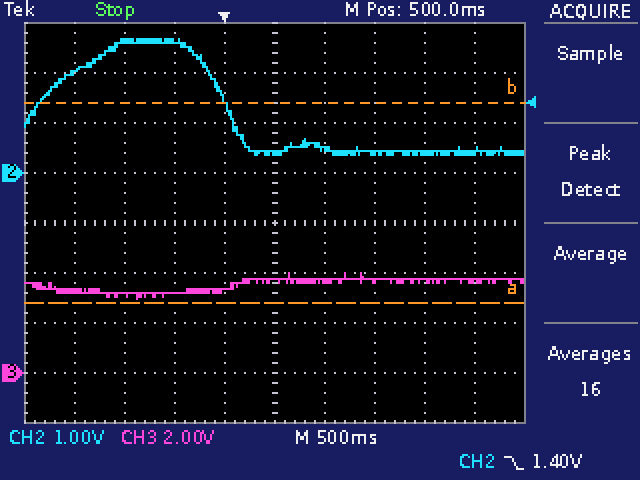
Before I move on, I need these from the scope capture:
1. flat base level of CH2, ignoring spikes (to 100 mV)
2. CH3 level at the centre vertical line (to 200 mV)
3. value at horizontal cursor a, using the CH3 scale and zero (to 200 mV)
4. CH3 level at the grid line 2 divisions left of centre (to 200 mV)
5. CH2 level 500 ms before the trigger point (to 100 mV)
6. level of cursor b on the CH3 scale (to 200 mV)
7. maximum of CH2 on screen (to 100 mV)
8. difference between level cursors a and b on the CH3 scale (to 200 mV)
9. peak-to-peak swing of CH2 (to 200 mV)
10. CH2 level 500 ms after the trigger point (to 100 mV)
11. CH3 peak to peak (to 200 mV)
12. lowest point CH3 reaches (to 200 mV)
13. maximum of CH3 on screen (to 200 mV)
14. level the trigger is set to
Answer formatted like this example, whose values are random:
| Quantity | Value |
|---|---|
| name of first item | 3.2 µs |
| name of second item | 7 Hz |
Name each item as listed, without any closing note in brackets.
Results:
| Quantity | Value |
|---|---|
| flat base level of CH2, ignoring spikes | 400 mV |
| CH3 level at the centre vertical line | 3.8 V |
| value at horizontal cursor a, using the CH3 scale and zero | 2.8 V |
| CH3 level at the grid line 2 divisions left of centre | 3.2 V |
| CH2 level 500 ms before the trigger point | 2.6 V |
| level of cursor b on the CH3 scale | 10.8 V |
| maximum of CH2 on screen | 2.7 V |
| difference between level cursors a and b on the CH3 scale | 8.0 V |
| peak-to-peak swing of CH2 | 2.4 V |
| CH2 level 500 ms after the trigger point | 400 mV |
| CH3 peak to peak | 1.0 V |
| lowest point CH3 reaches | 3.0 V |
| maximum of CH3 on screen | 4.0 V |
| level the trigger is set to | 1.40 V |
